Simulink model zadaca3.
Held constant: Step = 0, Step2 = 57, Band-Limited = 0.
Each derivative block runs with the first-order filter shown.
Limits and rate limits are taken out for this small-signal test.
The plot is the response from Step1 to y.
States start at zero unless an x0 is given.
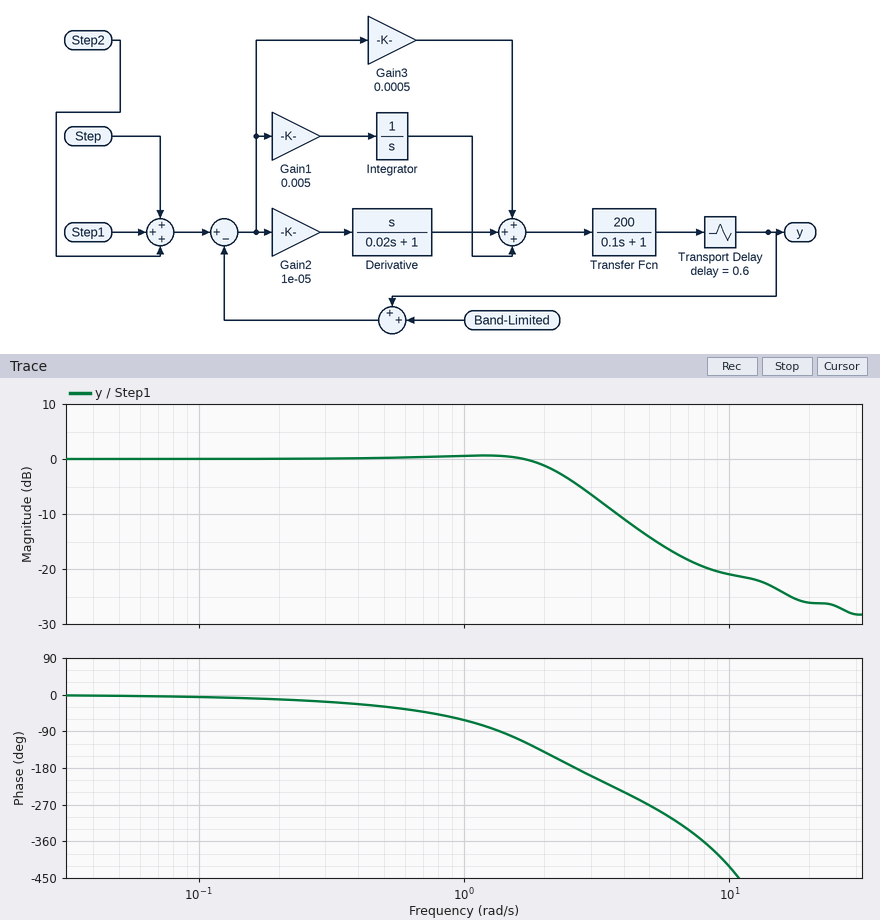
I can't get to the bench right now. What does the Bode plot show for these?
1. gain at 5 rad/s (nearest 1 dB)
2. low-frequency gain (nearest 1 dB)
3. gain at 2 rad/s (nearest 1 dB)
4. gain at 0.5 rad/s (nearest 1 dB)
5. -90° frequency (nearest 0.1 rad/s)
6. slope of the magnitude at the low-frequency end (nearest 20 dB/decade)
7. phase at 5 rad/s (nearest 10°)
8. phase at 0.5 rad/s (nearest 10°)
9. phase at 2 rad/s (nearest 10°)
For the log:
-14 dB
0 dB
-1 dB
0 dB
1.4 rad/s
0 dB/decade
-270°
-30°
-140°
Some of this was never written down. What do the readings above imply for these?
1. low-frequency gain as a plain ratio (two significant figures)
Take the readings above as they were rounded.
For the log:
1.0
